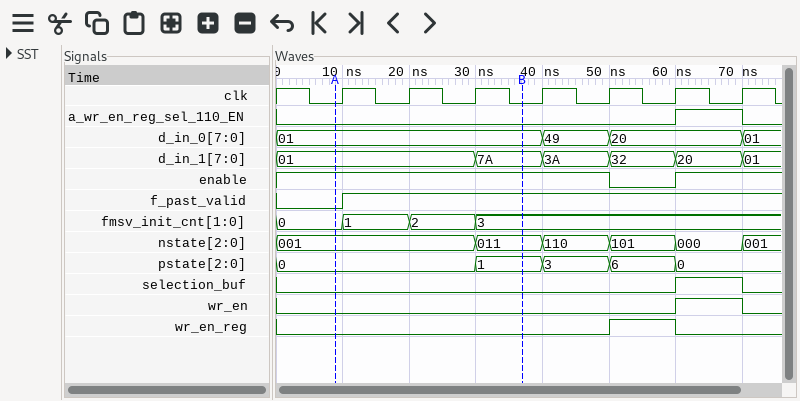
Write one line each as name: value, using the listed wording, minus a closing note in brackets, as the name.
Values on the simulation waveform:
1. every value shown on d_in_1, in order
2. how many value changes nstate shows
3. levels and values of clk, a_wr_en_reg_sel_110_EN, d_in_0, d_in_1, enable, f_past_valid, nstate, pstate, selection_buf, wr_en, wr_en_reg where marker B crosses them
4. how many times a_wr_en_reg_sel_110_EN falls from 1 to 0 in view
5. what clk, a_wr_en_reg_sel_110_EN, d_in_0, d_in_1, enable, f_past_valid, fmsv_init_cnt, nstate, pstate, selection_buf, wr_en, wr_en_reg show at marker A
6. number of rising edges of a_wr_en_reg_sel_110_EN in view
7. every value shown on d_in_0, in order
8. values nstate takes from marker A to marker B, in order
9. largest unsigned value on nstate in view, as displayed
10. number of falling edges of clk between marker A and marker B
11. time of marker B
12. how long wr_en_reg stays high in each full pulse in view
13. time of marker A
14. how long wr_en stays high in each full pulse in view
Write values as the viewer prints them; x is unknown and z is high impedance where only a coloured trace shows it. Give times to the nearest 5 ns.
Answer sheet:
every value shown on d_in_1, in order: 01, 7A, 3A, 32, 20, 01
how many value changes nstate shows: 5
levels and values of clk, a_wr_en_reg_sel_110_EN, d_in_0, d_in_1, enable, f_past_valid, nstate, pstate, selection_buf, wr_en, wr_en_reg where marker B crosses them: clk=0, a_wr_en_reg_sel_110_EN=0, d_in_0=01, d_in_1=7A, enable=1, f_past_valid=1, nstate=011, pstate=1, selection_buf=0, wr_en=0, wr_en_reg=0
how many times a_wr_en_reg_sel_110_EN falls from 1 to 0 in view: 1
what clk, a_wr_en_reg_sel_110_EN, d_in_0, d_in_1, enable, f_past_valid, fmsv_init_cnt, nstate, pstate, selection_buf, wr_en, wr_en_reg show at marker A: clk=0, a_wr_en_reg_sel_110_EN=0, d_in_0=01, d_in_1=01, enable=1, f_past_valid=0, fmsv_init_cnt=0, nstate=001, pstate=0, selection_buf=0, wr_en=0, wr_en_reg=0
number of rising edges of a_wr_en_reg_sel_110_EN in view: 1
every value shown on d_in_0, in order: 01, 49, 20, 01
values nstate takes from marker A to marker B, in order: 001, 011
largest unsigned value on nstate in view, as displayed: 110
number of falling edges of clk between marker A and marker B: 3
time of marker B: 35 ns
how long wr_en_reg stays high in each full pulse in view: 10 ns
time of marker A: 10 ns
how long wr_en stays high in each full pulse in view: 10 ns
